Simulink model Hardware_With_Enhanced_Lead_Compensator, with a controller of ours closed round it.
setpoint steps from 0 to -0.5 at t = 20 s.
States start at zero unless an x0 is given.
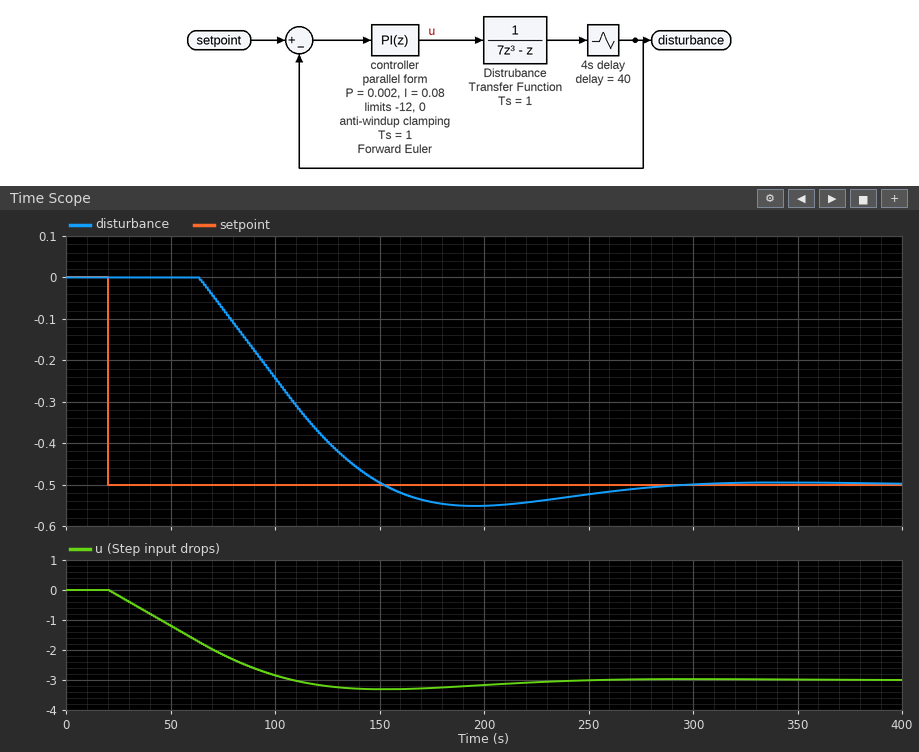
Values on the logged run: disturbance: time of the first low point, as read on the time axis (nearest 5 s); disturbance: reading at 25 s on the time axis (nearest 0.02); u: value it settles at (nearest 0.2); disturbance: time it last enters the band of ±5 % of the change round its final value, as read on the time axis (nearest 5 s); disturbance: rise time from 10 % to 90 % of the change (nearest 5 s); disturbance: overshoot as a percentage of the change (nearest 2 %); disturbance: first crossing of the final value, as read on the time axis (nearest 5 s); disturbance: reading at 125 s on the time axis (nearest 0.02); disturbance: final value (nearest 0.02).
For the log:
195 s
0.00
-3.0
250 s
65 s
10 %
150 s
-0.40
-0.50
